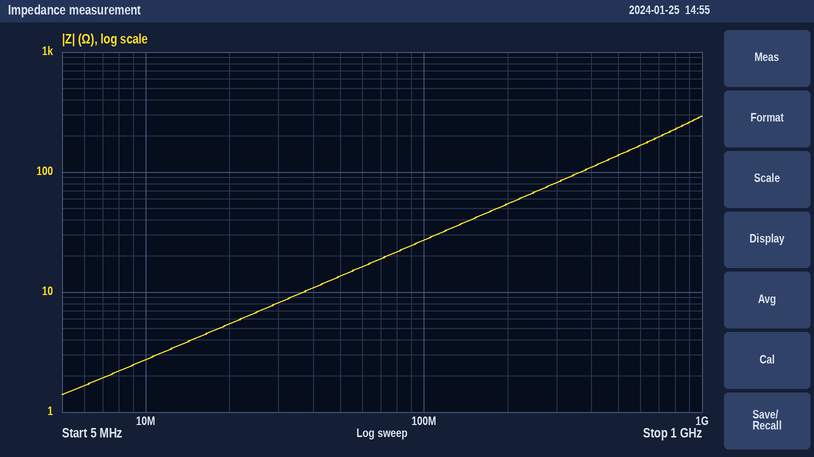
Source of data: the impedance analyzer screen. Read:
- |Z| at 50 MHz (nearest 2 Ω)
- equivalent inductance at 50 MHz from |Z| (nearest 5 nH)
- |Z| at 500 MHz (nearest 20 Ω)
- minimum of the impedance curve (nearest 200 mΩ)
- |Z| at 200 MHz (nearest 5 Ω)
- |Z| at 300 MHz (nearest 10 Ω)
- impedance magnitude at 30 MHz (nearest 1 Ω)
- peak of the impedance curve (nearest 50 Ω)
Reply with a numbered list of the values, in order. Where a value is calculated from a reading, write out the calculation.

1. 14 Ω
2. L = 14 Ω/(2π × 50 MHz) ≈ 45 nH
3. 140 Ω
4. 1.4 Ω
5. 55 Ω
6. 80 Ω
7. 8 Ω
8. 300 Ω
